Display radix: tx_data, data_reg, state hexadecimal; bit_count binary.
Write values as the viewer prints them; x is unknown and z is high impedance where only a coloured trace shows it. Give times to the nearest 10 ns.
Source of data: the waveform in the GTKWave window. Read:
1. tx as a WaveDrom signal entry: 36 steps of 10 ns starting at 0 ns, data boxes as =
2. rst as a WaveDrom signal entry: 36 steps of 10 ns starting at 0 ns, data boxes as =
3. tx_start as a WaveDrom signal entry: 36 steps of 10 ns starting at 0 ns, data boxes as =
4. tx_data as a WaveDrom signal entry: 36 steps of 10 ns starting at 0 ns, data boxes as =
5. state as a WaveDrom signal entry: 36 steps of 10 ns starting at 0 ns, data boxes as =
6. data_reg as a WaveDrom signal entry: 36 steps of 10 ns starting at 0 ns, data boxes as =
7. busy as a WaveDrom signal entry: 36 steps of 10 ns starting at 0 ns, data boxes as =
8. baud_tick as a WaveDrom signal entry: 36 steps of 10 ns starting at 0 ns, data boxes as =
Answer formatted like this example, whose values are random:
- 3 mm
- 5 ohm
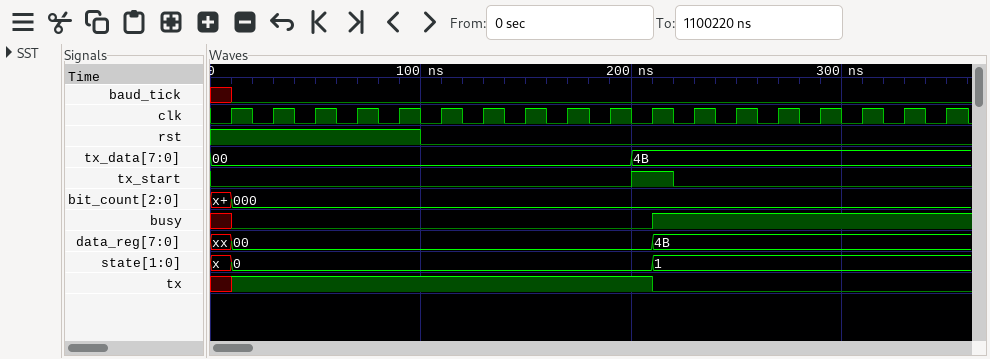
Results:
- {name: 'tx', wave: 'x1...................0..............'}
- {name: 'rst', wave: '1.........0.........................'}
- {name: 'tx_start', wave: '0...................1.0.............'}
- {name: 'tx_data', wave: '=...................=...............', data: '00 4B'}
- {name: 'state', wave: 'x=...................=..............', data: '0 1'}
- {name: 'data_reg', wave: 'x=...................=..............', data: '00 4B'}
- {name: 'busy', wave: 'x0...................1..............'}
- {name: 'baud_tick', wave: 'x0..................................'}
